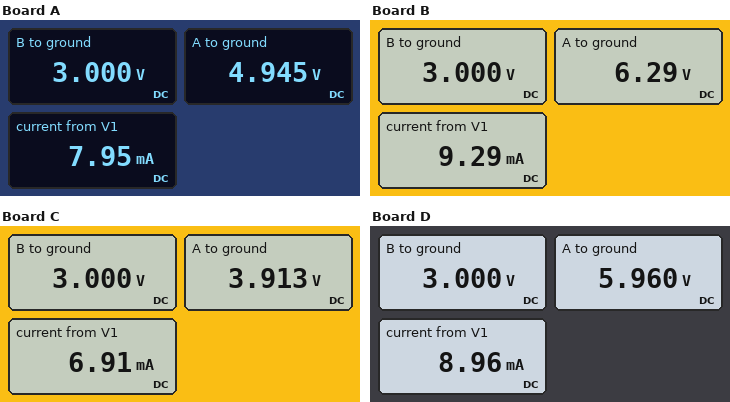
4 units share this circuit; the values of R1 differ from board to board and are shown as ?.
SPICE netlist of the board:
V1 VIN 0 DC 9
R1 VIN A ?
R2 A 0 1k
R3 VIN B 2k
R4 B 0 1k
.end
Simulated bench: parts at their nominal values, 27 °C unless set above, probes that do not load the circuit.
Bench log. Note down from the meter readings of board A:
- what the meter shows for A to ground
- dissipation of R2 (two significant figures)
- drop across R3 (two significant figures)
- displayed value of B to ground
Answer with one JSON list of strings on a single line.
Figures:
["4.945 V", "24 mW", "6.0 V", "3.000 V"]
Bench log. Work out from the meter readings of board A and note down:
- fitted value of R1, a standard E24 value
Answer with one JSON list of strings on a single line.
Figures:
["820 Ω"]
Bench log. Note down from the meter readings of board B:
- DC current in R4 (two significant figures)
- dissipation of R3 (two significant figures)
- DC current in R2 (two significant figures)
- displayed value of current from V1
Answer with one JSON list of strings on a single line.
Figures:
["3.0 mA", "18 mW", "6.3 mA", "9.29 mA"]
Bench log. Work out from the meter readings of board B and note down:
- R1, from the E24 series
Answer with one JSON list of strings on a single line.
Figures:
["430 Ω"]
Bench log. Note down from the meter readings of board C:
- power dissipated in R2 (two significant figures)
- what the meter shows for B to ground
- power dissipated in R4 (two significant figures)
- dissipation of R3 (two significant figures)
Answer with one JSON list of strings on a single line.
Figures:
["15 mW", "3.000 V", "9.0 mW", "18 mW"]
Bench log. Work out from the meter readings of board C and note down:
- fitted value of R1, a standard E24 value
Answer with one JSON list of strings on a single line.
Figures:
["1.3 kΩ"]
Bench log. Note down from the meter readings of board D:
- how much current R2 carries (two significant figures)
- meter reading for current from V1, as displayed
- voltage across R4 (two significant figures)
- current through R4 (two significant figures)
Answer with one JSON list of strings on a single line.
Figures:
["6.0 mA", "8.96 mA", "3.0 V", "3.0 mA"]
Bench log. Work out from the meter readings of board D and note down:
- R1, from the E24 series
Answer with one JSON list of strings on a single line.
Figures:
["510 Ω"]
